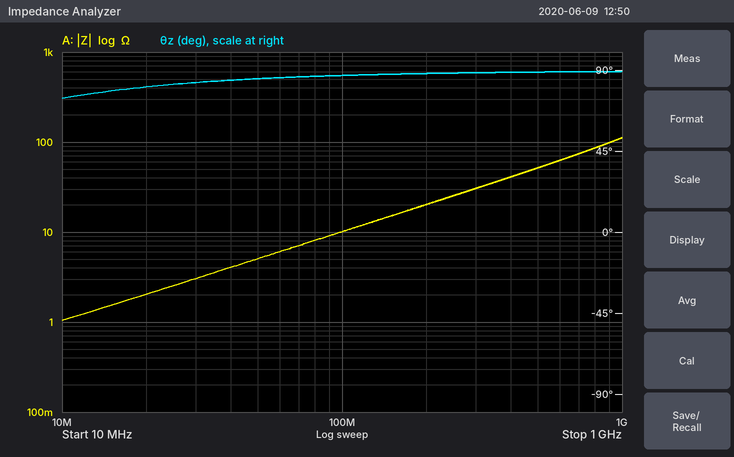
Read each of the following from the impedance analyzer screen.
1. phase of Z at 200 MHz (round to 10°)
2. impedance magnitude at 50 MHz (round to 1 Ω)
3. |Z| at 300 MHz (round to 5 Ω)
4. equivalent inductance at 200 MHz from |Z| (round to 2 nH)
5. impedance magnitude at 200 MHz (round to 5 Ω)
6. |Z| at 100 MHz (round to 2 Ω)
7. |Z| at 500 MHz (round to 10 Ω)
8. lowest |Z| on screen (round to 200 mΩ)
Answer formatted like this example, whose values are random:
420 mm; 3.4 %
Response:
90°; 5 Ω; 30 Ω; 16 nH; 20 Ω; 10 Ω; 50 Ω; 1.0 Ω
